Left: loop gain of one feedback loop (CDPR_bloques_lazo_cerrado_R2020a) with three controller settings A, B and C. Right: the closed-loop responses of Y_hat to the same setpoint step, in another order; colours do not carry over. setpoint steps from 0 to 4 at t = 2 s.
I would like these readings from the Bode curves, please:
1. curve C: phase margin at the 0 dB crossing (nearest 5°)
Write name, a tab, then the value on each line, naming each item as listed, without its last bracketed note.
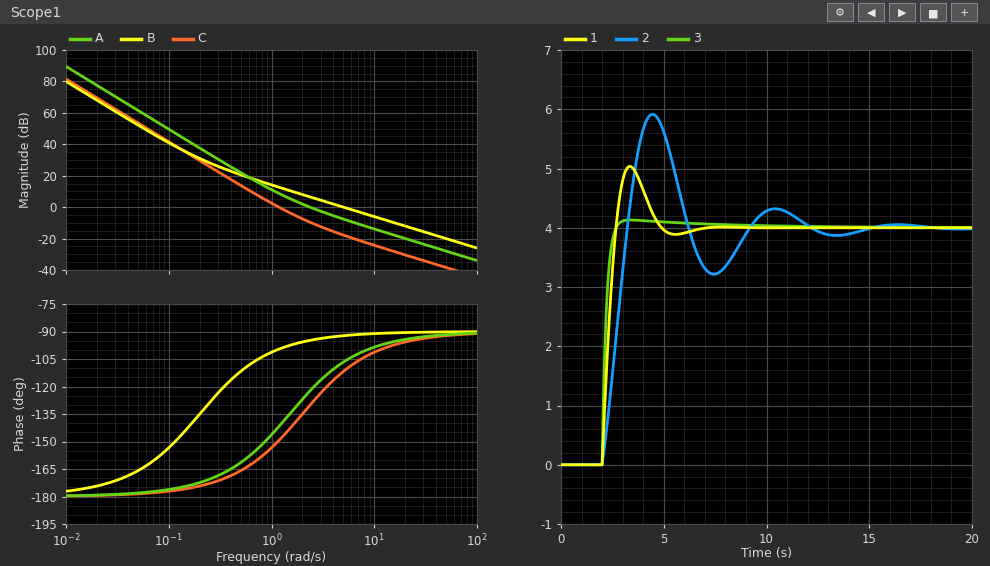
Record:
curve C: phase margin at the 0 dB crossing	30°
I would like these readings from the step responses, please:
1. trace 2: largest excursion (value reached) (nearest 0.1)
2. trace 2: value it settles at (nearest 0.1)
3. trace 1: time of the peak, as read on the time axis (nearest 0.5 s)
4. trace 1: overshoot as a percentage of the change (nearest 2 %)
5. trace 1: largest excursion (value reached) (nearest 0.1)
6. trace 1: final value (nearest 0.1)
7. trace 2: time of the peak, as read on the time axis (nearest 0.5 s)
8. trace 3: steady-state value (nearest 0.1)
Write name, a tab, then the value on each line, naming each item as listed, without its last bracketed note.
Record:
trace 2: largest excursion (value reached)	5.9
trace 2: value it settles at	4.0
trace 1: time of the peak, as read on the time axis	3.5 s
trace 1: overshoot as a percentage of the change	26 %
trace 1: largest excursion (value reached)	5.0
trace 1: final value	4.0
trace 2: time of the peak, as read on the time axis	4.5 s
trace 3: steady-state value	4.0
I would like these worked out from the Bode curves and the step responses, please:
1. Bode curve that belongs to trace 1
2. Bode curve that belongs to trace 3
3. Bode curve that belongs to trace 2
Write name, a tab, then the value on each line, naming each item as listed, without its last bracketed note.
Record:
Bode curve that belongs to trace 1	A
Bode curve that belongs to trace 3	B
Bode curve that belongs to trace 2	C
